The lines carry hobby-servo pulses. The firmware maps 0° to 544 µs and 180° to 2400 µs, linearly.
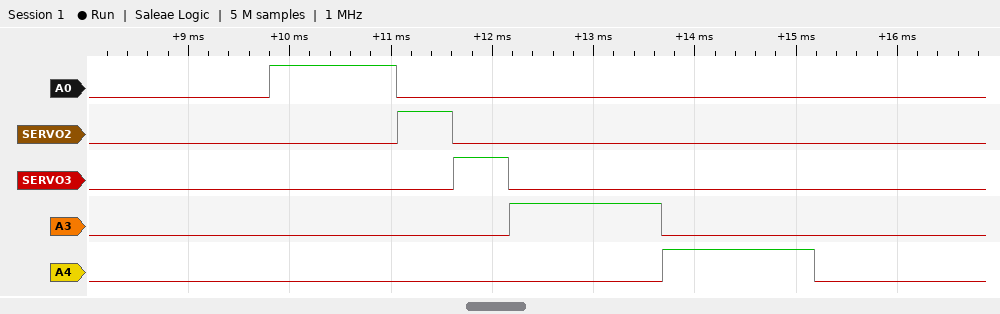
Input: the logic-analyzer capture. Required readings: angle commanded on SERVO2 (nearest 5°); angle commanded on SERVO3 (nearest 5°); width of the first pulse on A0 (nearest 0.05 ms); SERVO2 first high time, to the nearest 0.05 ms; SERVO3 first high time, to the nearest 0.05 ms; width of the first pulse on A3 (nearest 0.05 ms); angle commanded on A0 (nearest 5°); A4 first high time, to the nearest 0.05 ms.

0°
0°
1.25 ms
0.55 ms
0.55 ms
1.50 ms
70°
1.50 ms
